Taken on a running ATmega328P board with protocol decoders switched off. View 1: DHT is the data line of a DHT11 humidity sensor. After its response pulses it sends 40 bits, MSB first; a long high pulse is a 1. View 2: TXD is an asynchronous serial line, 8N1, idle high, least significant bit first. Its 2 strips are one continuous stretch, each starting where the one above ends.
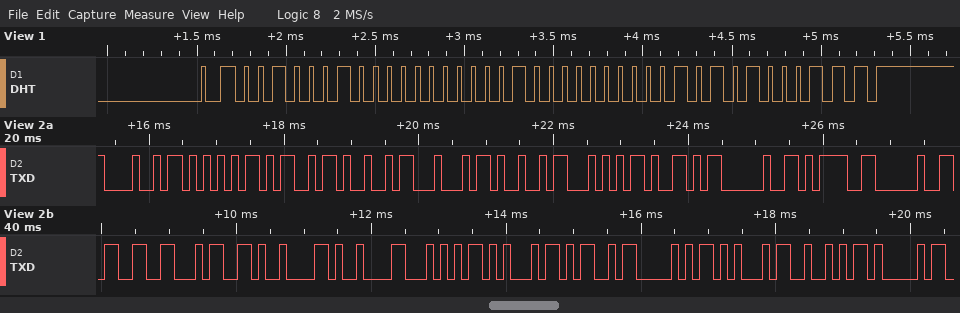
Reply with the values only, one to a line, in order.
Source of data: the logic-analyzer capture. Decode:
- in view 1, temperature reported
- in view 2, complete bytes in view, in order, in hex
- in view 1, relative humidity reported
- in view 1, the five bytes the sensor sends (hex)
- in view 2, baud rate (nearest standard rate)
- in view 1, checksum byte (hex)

32.5 °C
48 55 4D 49 44 49 54 59 20 3D 20 33 34 09 09 54 45 4D 50 45 52 41
34 %
22 00 20 05 47
9600 baud
0x47
